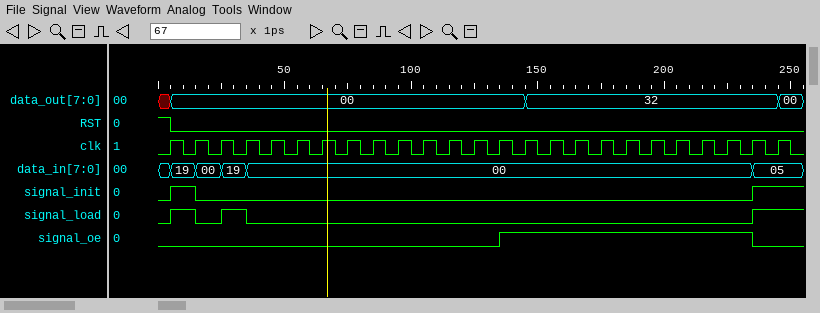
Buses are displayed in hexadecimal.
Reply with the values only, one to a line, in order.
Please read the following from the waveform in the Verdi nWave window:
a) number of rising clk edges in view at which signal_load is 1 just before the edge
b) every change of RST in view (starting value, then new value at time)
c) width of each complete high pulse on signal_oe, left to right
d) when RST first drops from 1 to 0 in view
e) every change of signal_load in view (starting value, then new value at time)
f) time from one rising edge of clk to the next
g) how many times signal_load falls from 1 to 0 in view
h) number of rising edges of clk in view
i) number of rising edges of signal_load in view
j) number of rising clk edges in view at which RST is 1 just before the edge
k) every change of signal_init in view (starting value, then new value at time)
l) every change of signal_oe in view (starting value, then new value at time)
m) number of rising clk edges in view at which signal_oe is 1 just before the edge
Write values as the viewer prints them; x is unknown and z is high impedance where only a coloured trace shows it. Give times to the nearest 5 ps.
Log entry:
3
1, 0 at 5 ps
100 ps
5 ps
0, 1 at 5 ps, 0 at 15 ps, 1 at 25 ps, 0 at 35 ps, 1 at 235 ps
10 ps
2
25
3
1
0, 1 at 5 ps, 0 at 15 ps, 1 at 235 ps
0, 1 at 135 ps, 0 at 235 ps
10
